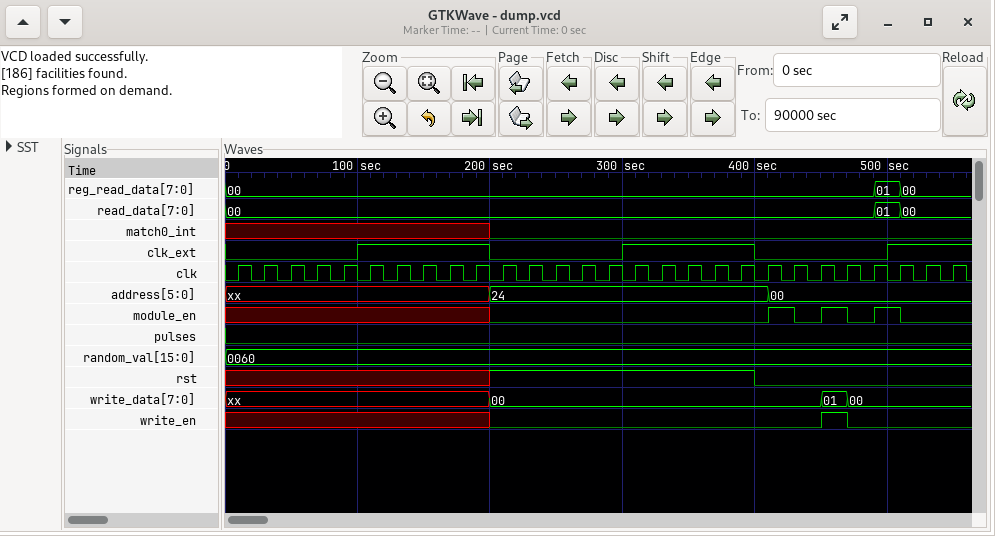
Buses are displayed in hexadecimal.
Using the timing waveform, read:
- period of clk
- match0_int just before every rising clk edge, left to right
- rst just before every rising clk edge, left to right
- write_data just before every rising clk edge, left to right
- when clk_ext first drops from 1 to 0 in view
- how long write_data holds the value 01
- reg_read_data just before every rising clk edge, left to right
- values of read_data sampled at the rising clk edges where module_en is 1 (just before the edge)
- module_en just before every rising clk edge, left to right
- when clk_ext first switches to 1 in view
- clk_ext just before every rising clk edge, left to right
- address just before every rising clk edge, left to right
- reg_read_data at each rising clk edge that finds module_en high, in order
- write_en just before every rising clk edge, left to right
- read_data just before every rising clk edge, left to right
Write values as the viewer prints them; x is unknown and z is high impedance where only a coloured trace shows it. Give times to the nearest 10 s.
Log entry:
20 s
x x x x x x x x x x 0 0 0 0 0 0 0 0 0 0 0 0 0 0 0 0 0 0
x x x x x x x x x x 1 1 1 1 1 1 1 1 1 1 0 0 0 0 0 0 0 0
xx, xx, xx, xx, xx, xx, xx, xx, xx, xx, 00, 00, 00, 00, 00, 00, 00, 00, 00, 00, 00, 00, 00, 01, 00, 00, 00, 00
200 s
20 s
00, 00, 00, 00, 00, 00, 00, 00, 00, 00, 00, 00, 00, 00, 00, 00, 00, 00, 00, 00, 00, 00, 00, 00, 00, 01, 00, 00
00, 00, 01
x x x x x x x x x x 0 0 0 0 0 0 0 0 0 0 0 1 0 1 0 1 0 0
100 s
0 0 0 0 0 1 1 1 1 1 0 0 0 0 0 1 1 1 1 1 0 0 0 0 0 1 1 1
xx, xx, xx, xx, xx, xx, xx, xx, xx, xx, 24, 24, 24, 24, 24, 24, 24, 24, 24, 24, 24, 00, 00, 00, 00, 00, 00, 00
00, 00, 01
x x x x x x x x x x 0 0 0 0 0 0 0 0 0 0 0 0 0 1 0 0 0 0
00, 00, 00, 00, 00, 00, 00, 00, 00, 00, 00, 00, 00, 00, 00, 00, 00, 00, 00, 00, 00, 00, 00, 00, 00, 01, 00, 00
